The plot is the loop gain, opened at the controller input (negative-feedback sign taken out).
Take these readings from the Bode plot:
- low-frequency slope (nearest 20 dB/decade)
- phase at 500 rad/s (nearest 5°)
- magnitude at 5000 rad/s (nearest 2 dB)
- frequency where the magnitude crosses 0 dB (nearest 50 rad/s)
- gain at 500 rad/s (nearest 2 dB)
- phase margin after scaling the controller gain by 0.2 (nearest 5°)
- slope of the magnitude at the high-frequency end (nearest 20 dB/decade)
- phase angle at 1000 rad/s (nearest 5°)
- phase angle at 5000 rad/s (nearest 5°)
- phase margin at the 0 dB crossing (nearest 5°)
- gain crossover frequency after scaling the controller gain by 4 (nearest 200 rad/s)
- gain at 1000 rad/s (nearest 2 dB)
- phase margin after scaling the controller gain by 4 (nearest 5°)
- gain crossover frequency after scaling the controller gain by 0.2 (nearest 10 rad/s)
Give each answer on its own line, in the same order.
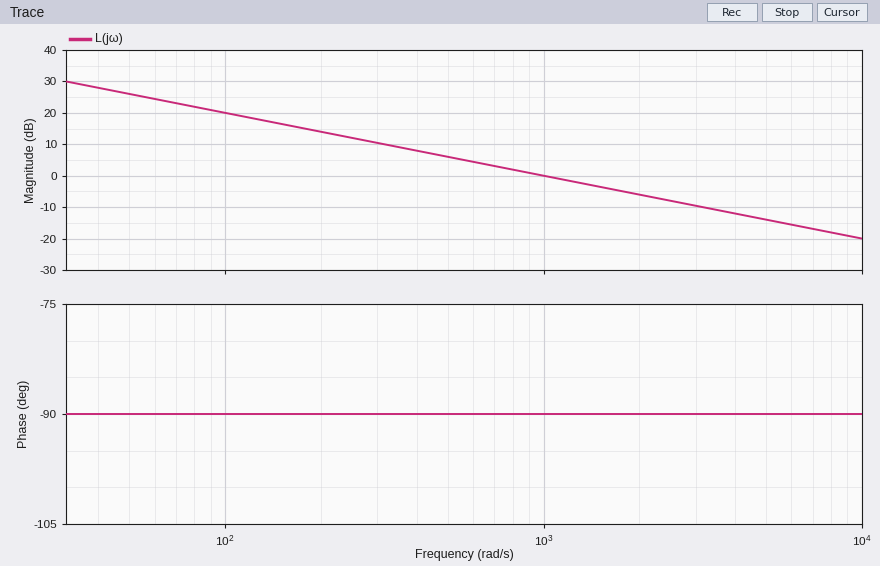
-20 dB/decade
-90°
-14 dB
1000 rad/s
6 dB
90°
-20 dB/decade
-90°
-90°
90°
4000 rad/s
0 dB
90°
200 rad/s
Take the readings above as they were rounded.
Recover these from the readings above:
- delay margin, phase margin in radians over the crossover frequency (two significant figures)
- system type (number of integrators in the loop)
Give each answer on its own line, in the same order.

0.0016 s
1
